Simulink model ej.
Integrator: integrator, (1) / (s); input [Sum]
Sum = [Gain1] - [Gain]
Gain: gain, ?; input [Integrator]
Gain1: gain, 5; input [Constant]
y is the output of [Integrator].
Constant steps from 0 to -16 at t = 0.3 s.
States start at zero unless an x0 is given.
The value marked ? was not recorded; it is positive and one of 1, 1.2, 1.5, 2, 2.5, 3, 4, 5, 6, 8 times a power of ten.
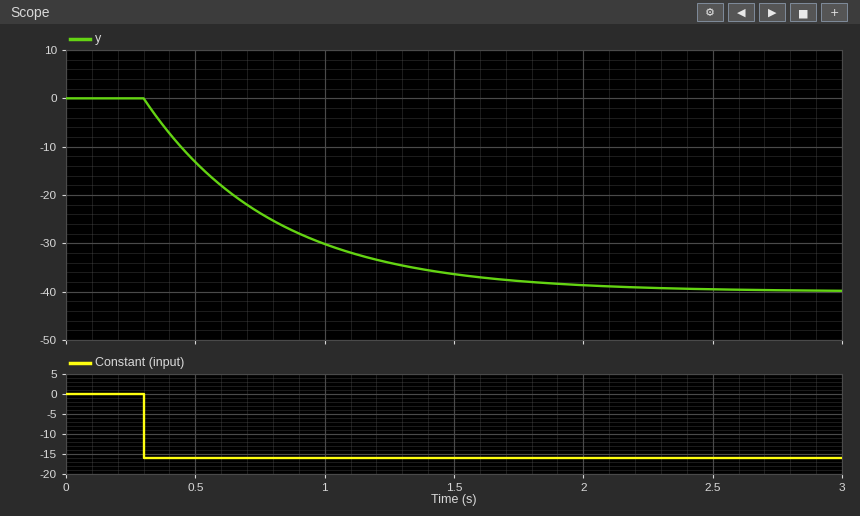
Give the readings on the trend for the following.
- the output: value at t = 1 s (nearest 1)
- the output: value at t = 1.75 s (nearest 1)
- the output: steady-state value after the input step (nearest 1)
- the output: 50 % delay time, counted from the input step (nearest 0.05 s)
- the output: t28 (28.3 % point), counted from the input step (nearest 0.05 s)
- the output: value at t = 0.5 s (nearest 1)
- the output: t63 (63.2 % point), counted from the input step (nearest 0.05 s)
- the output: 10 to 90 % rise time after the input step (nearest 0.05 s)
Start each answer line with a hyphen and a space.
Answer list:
- -30
- -38
- -40
- 0.35 s
- 0.15 s
- -13
- 0.50 s
- 1.10 s
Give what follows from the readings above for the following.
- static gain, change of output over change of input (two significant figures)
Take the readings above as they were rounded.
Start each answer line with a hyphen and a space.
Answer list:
- 2.5
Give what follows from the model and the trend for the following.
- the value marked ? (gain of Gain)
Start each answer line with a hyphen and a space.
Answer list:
- 2
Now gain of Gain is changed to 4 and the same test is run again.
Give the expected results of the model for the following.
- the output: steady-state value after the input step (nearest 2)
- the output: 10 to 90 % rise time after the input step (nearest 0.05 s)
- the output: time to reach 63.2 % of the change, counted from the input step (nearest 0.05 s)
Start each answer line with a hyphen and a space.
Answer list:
- -20
- 0.55 s
- 0.25 s
